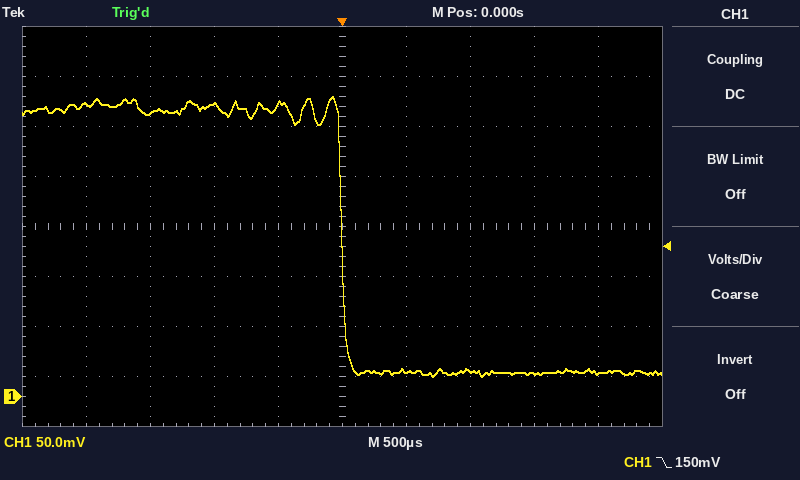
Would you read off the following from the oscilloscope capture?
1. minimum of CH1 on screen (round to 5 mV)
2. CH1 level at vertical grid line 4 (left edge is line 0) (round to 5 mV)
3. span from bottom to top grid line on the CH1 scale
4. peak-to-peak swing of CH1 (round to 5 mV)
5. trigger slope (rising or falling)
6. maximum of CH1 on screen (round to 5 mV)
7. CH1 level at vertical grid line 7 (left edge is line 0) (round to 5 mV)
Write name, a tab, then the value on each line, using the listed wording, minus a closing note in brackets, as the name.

minimum of CH1 on screen	20 mV
CH1 level at vertical grid line 4 (left edge is line 0)	290 mV
span from bottom to top grid line on the CH1 scale	400 mV
peak-to-peak swing of CH1	280 mV
trigger slope	falling
maximum of CH1 on screen	300 mV
CH1 level at vertical grid line 7 (left edge is line 0)	25 mV
